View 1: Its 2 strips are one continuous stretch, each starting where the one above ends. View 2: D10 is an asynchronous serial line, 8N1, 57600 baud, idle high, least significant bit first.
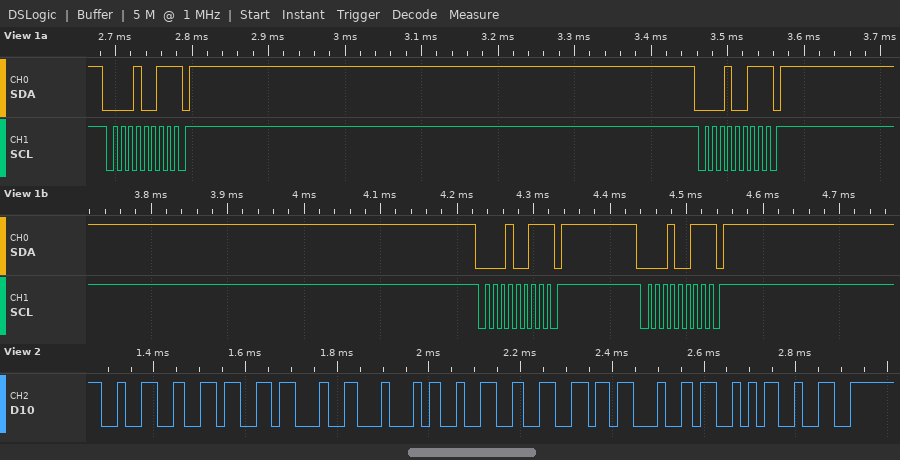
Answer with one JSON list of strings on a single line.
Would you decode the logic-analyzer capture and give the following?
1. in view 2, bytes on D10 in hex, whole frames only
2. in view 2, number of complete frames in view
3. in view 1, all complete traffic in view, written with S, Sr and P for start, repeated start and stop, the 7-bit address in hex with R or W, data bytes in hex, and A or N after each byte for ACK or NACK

["32 36 23 44 32 66 23 53 32", "9", "S 09R N P S 09R N P S 09R N P S 09R N P"]
